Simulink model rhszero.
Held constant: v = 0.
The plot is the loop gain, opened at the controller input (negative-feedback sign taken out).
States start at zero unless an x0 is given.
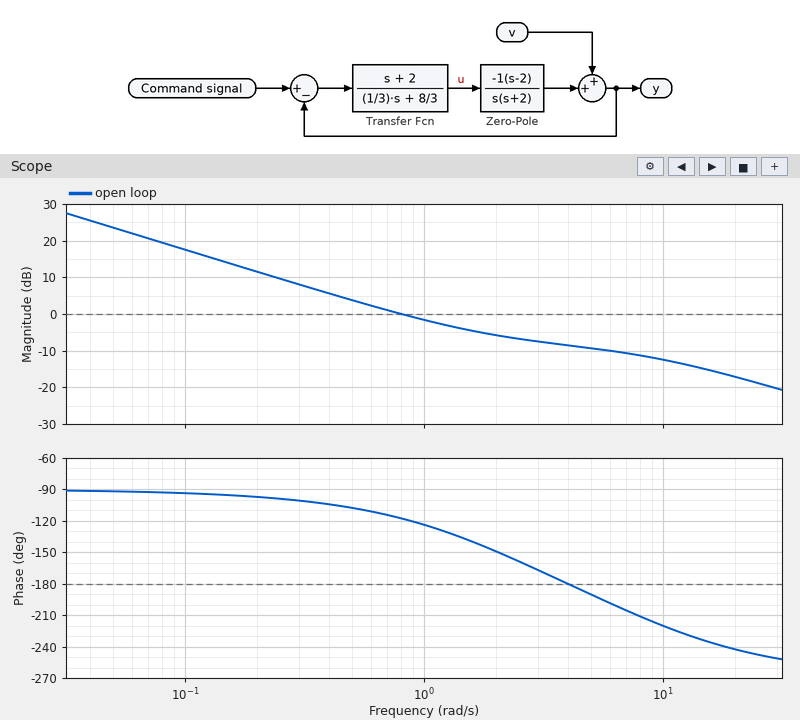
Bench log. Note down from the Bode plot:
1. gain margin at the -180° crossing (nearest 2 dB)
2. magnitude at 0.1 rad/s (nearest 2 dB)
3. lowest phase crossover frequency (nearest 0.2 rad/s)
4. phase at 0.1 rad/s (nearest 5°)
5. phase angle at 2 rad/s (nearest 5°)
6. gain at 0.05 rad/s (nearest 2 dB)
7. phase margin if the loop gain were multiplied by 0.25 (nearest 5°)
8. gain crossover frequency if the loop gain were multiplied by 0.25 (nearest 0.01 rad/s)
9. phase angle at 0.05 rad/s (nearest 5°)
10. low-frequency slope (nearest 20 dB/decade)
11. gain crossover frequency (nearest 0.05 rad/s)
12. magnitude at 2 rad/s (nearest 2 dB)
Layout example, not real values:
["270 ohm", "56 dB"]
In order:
["8 dB", "18 dB", "4.0 rad/s", "-95°", "-150°", "24 dB", "85°", "0.19 rad/s", "-90°", "-20 dB/decade", "0.80 rad/s", "-6 dB"]
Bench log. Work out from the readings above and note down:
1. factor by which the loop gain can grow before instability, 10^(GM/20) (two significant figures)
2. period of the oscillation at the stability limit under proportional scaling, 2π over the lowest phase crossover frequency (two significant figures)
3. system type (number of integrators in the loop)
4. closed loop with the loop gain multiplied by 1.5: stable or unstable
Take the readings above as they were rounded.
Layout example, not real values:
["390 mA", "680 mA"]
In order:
["2.5", "1.6 s", "1", "stable"]
